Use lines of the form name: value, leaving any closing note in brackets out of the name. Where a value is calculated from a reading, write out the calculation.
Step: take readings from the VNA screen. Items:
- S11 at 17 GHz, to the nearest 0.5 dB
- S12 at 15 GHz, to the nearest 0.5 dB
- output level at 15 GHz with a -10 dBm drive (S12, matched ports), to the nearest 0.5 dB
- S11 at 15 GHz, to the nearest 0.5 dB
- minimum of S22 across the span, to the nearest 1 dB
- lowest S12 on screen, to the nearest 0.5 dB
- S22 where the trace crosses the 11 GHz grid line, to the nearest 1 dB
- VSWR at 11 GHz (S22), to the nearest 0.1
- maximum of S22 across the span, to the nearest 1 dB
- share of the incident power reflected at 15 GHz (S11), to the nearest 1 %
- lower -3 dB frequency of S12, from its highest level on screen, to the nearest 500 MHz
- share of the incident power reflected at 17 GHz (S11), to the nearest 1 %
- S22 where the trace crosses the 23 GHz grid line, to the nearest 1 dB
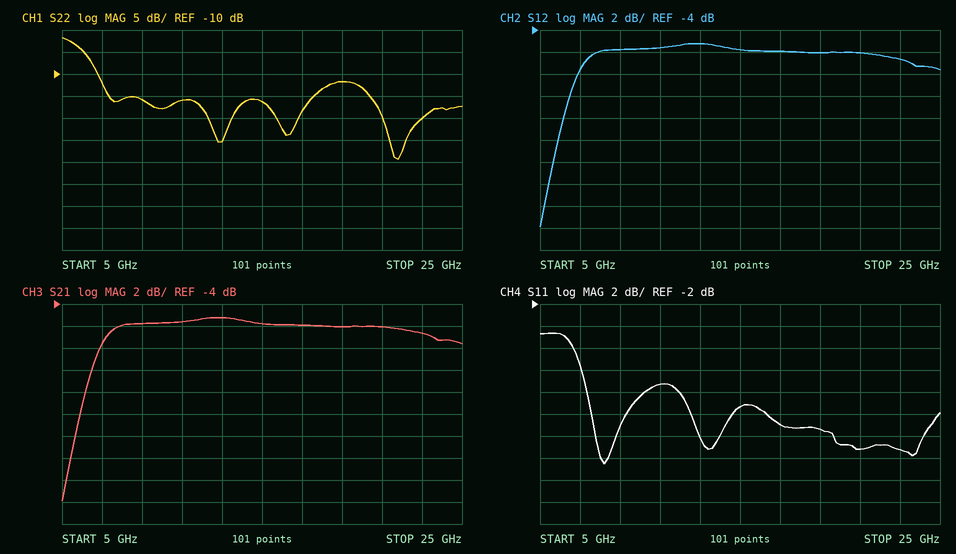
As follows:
S11 at 17 GHz, to the nearest 0.5 dB: -13.0 dB
S12 at 15 GHz, to the nearest 0.5 dB: -6.0 dB
output level at 15 GHz with a -10 dBm drive (S12, matched ports), to the nearest 0.5 dB: -10 dBm + (-6.0 dB) = -16.0 dBm
S11 at 15 GHz, to the nearest 0.5 dB: -11.5 dB
minimum of S22 across the span, to the nearest 1 dB: -29 dB
lowest S12 on screen, to the nearest 0.5 dB: -22.0 dB
S22 where the trace crosses the 11 GHz grid line, to the nearest 1 dB: -16 dB
VSWR at 11 GHz (S22), to the nearest 0.1: |Γ| = 10^(-16/20) = 0.1585; VSWR = (1 + 0.1585)/(1 − 0.1585) ≈ 1.4
maximum of S22 across the span, to the nearest 1 dB: -2 dB
share of the incident power reflected at 15 GHz (S11), to the nearest 1 %: 10^(-11.5/10) ≈ 7 %
lower -3 dB frequency of S12, from its highest level on screen, to the nearest 500 MHz: 7.0 GHz
share of the incident power reflected at 17 GHz (S11), to the nearest 1 %: 10^(-13/10) ≈ 5 %
S22 where the trace crosses the 23 GHz grid line, to the nearest 1 dB: -20 dB
